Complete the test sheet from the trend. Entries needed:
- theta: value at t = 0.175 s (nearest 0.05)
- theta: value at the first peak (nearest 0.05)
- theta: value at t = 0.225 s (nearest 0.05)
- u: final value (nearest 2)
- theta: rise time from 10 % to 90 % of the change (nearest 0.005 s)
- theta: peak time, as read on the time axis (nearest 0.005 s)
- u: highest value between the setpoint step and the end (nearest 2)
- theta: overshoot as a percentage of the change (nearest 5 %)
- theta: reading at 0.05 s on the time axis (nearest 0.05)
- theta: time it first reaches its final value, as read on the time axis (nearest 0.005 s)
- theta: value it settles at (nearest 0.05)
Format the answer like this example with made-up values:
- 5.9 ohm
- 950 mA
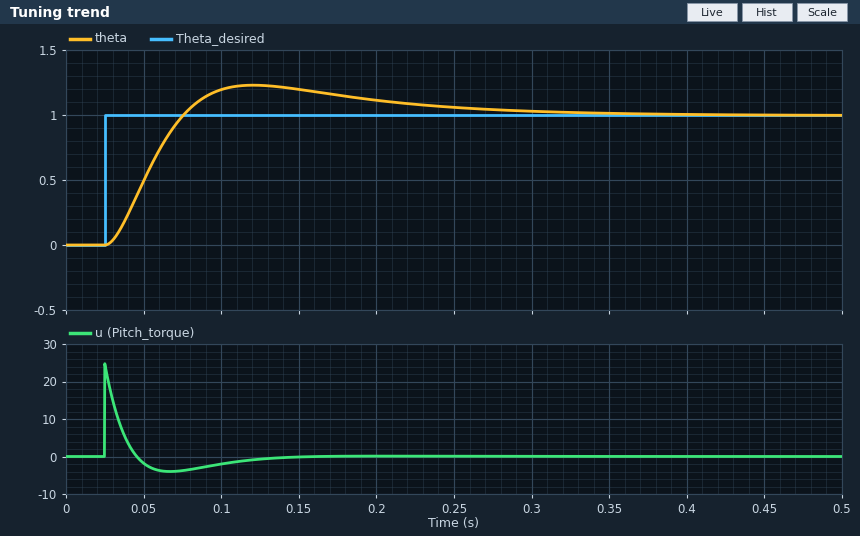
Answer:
- 1.15
- 1.25
- 1.10
- 0
- 0.035 s
- 0.120 s
- 24
- 25 %
- 0.50
- 0.075 s
- 1.00
